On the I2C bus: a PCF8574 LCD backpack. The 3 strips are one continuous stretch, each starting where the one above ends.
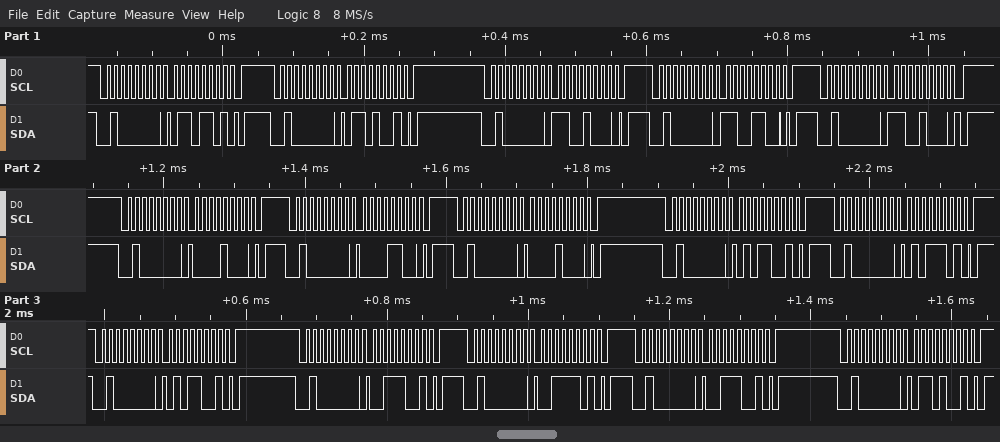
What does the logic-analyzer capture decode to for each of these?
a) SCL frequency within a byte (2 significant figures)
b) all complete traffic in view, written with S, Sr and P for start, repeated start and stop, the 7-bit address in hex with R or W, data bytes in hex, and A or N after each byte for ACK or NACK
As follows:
100 kHz
S 20W A 6D A P S 20W A 69 A P S 20W A C8 A P S 20W A CC A P S 20W A C8 A P S 20W A 08 A P S 20W A 0C A P S 20W A 08 A P S 20W A 59 A P S 20W A 5D A P S 20W A 59 A P S 20W A 39 A P S 20W A 3D A P S 20W A 39 A P S 20W A 69 A P
